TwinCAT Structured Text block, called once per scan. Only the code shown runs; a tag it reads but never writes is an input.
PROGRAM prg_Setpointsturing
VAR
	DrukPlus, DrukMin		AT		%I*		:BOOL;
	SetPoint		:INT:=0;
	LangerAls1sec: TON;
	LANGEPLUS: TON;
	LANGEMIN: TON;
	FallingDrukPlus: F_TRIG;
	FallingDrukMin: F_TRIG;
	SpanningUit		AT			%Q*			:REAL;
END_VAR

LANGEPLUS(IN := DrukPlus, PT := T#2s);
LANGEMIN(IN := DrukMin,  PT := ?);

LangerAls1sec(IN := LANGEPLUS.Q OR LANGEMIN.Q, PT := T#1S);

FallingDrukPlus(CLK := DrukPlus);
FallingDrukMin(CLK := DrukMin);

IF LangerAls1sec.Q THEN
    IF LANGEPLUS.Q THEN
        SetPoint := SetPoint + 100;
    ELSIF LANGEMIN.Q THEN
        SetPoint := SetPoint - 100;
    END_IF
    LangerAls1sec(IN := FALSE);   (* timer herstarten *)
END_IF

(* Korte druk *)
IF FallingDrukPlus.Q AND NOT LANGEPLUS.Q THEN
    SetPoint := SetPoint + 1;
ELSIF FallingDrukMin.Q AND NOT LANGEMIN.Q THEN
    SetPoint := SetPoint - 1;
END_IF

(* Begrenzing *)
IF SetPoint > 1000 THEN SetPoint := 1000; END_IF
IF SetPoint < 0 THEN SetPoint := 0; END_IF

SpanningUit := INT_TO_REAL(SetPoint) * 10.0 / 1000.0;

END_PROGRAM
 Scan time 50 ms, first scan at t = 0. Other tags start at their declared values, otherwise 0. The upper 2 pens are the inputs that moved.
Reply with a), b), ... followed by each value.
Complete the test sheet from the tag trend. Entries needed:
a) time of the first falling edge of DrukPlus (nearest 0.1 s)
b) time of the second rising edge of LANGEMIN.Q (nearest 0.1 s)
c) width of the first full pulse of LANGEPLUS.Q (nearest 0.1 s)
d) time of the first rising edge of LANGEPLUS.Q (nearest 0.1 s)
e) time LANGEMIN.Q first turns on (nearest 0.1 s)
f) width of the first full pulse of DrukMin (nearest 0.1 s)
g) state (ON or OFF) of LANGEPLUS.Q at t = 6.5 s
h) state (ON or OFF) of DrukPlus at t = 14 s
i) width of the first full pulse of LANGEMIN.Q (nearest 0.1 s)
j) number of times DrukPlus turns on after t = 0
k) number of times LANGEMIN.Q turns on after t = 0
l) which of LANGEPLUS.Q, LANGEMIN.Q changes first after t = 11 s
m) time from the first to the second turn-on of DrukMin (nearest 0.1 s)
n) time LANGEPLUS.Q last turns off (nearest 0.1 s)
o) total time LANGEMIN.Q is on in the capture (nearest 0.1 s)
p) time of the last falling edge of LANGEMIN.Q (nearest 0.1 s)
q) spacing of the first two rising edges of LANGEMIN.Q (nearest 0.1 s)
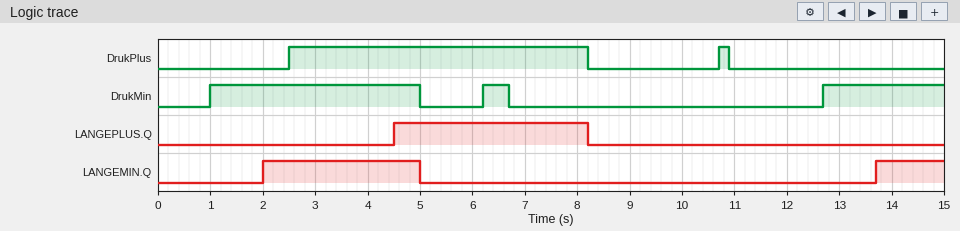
a) 8.2 s
b) 13.7 s
c) 3.7 s
d) 4.5 s
e) 2.0 s
f) 4.0 s
g) ON
h) OFF
i) 3.0 s
j) 2
k) 2
l) LANGEMIN.Q
m) 5.2 s
n) 8.2 s
o) 4.3 s
p) 5.0 s
q) 11.7 s
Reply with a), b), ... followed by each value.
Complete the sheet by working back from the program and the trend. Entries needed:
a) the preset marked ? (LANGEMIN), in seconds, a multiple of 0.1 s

a) 1.0 s
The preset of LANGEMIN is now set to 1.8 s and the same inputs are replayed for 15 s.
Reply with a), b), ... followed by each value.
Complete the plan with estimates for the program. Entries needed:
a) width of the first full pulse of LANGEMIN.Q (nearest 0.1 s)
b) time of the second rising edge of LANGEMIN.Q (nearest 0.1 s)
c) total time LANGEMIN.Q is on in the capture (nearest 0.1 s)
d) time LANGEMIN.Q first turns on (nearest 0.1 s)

a) 2.2 s
b) 14.5 s
c) 2.7 s
d) 2.8 s
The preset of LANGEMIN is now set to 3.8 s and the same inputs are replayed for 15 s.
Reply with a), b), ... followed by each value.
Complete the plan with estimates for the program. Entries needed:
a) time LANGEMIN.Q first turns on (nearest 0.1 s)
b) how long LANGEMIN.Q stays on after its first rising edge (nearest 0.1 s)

a) 4.8 s
b) 0.2 s
